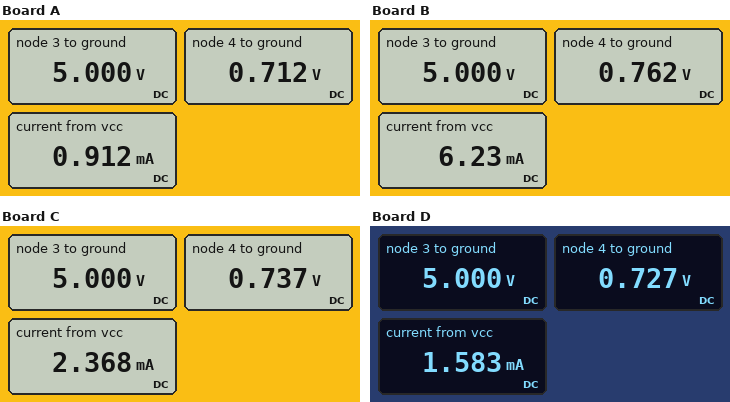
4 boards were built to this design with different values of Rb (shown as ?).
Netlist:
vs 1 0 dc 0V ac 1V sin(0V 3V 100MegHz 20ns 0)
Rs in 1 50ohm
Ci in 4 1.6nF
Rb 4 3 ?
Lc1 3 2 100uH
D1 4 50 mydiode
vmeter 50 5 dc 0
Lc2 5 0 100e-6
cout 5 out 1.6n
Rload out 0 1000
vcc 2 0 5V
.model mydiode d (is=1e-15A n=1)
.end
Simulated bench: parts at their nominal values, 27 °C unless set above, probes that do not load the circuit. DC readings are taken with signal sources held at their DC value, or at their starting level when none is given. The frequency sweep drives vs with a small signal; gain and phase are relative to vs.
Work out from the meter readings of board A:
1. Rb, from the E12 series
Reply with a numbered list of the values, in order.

1. 4.7 kΩ
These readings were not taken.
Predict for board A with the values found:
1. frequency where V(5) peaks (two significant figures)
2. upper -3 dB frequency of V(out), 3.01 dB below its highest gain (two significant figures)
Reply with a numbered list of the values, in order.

1. 410 kHz
2. 730 kHz
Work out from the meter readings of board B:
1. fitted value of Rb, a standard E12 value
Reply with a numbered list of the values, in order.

1. 680 Ω
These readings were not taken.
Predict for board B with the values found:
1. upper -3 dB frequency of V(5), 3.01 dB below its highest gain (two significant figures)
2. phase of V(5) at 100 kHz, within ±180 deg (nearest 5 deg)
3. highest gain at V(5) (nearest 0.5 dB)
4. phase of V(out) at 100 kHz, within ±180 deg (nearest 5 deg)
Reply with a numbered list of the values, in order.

1. 4.2 MHz
2. 170 deg
3. 2.5 dB
4. -145 deg
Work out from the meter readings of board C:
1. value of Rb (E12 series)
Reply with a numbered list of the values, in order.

1. 1.8 kΩ
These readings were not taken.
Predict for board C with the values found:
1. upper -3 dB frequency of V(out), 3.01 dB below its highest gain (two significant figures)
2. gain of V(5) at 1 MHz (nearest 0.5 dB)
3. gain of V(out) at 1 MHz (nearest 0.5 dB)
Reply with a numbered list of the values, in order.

1. 790 kHz
2. 0.5 dB
3. 0.5 dB
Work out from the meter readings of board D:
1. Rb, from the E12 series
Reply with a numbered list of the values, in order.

1. 2.7 kΩ
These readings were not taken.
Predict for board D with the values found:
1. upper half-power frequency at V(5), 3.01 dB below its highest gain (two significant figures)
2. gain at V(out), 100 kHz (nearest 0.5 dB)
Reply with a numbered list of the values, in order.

1. 700 kHz
2. -26.0 dB
